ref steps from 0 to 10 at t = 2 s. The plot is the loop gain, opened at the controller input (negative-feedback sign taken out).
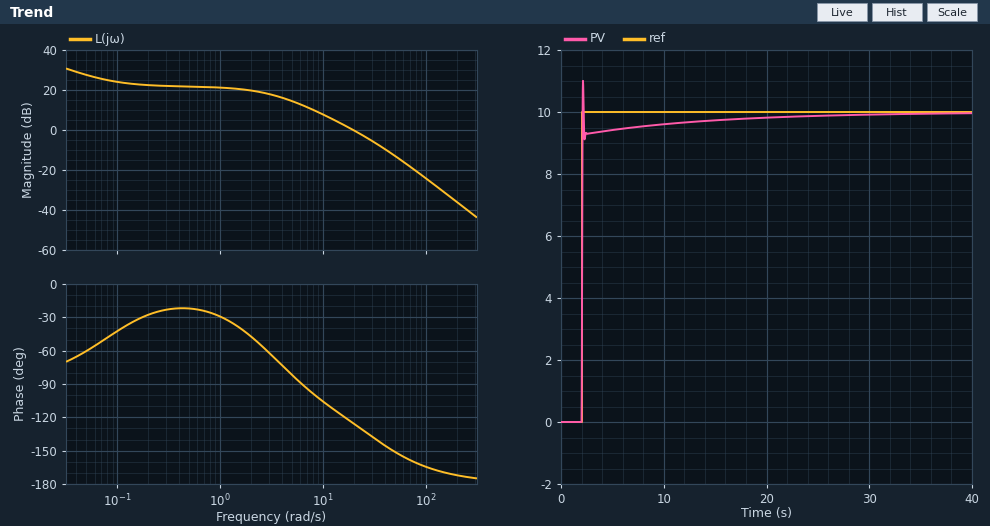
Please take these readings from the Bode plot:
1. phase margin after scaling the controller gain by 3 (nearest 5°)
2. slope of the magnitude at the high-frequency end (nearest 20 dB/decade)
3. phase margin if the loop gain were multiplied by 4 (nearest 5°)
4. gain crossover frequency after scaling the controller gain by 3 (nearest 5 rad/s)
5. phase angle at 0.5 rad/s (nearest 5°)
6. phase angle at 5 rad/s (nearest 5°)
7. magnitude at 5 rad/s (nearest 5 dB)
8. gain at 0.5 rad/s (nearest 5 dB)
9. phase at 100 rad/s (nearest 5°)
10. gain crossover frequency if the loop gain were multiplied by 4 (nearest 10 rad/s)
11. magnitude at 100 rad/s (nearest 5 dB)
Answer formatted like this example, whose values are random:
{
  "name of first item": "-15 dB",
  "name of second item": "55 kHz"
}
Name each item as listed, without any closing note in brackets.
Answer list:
{
  "phase margin after scaling the controller gain by 3": "35°",
  "slope of the magnitude at the high-frequency end": "-40 dB/decade",
  "phase margin if the loop gain were multiplied by 4": "30°",
  "gain crossover frequency after scaling the controller gain by 3": "40 rad/s",
  "phase angle at 0.5 rad/s": "-20°",
  "phase angle at 5 rad/s": "-80°",
  "magnitude at 5 rad/s": "15 dB",
  "gain at 0.5 rad/s": "20 dB",
  "phase at 100 rad/s": "-165°",
  "gain crossover frequency if the loop gain were multiplied by 4": "50 rad/s",
  "magnitude at 100 rad/s": "-25 dB"
}
